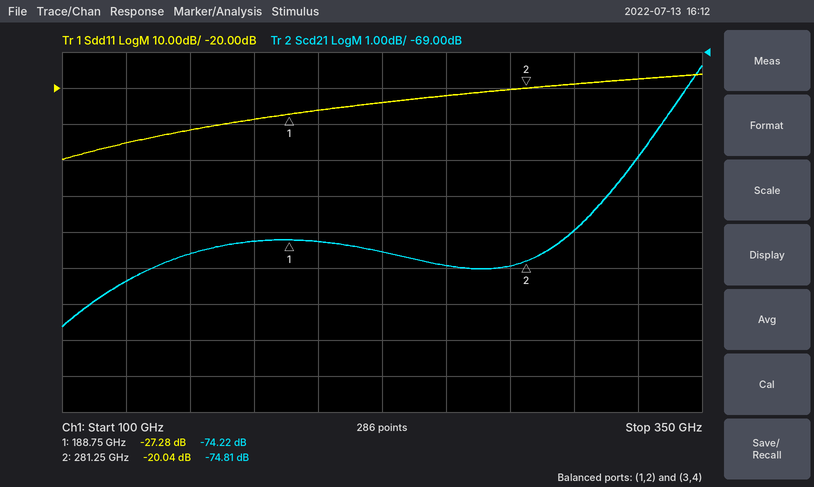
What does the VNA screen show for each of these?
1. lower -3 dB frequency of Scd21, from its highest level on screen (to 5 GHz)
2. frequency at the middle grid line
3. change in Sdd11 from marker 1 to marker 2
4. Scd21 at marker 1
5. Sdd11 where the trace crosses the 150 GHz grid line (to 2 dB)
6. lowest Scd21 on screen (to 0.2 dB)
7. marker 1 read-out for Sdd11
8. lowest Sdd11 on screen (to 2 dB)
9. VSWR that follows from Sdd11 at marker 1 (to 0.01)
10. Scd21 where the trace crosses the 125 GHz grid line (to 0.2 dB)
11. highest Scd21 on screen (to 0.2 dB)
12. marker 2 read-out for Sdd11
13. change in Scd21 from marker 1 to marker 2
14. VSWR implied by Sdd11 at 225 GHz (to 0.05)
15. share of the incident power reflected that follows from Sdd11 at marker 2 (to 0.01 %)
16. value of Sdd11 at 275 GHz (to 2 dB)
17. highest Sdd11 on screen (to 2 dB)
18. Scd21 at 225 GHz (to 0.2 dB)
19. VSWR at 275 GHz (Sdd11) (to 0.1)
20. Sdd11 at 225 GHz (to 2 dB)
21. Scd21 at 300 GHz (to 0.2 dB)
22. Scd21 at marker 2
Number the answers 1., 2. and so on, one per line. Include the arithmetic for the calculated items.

1. 320 GHz
2. 225 GHz
3. -20.04 − (-27.28) = 7.24 dB
4. -74.22 dB
5. -32 dB
6. -76.6 dB
7. -27.28 dB
8. -40 dB
9. (1 + 0.0433)/(1 − 0.0433) ≈ 1.09
10. -75.4 dB
11. -69.4 dB
12. -20.04 dB
13. -74.81 − (-74.22) = -0.59 dB
14. |Γ| = 10^(-24/20) = 0.0631; VSWR = (1 + 0.0631)/(1 − 0.0631) ≈ 1.13, so 1.15 to the nearest 0.05
15. 10^(-20.04/10) ≈ 0.99 %
16. -20 dB
17. -16 dB
18. -74.6 dB
19. |Γ| = 10^(-20/20) = 0.1000; VSWR = (1 + 0.1000)/(1 − 0.1000) ≈ 1.2
20. -24 dB
21. -74.0 dB
22. -74.81 dB
